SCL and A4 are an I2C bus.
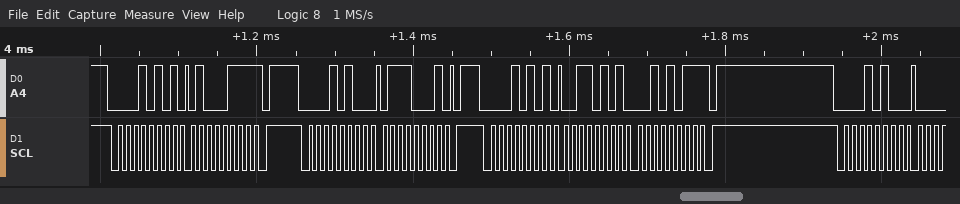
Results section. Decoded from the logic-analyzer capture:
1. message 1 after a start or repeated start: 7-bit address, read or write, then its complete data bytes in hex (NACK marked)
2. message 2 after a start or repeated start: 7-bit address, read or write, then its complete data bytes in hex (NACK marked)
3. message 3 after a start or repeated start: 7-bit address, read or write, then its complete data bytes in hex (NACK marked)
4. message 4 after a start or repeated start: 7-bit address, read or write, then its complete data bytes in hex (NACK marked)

0x0A read: 47 NACK
0x0A write: 71
0x0A read: 35 2B NACK
0x0A write
